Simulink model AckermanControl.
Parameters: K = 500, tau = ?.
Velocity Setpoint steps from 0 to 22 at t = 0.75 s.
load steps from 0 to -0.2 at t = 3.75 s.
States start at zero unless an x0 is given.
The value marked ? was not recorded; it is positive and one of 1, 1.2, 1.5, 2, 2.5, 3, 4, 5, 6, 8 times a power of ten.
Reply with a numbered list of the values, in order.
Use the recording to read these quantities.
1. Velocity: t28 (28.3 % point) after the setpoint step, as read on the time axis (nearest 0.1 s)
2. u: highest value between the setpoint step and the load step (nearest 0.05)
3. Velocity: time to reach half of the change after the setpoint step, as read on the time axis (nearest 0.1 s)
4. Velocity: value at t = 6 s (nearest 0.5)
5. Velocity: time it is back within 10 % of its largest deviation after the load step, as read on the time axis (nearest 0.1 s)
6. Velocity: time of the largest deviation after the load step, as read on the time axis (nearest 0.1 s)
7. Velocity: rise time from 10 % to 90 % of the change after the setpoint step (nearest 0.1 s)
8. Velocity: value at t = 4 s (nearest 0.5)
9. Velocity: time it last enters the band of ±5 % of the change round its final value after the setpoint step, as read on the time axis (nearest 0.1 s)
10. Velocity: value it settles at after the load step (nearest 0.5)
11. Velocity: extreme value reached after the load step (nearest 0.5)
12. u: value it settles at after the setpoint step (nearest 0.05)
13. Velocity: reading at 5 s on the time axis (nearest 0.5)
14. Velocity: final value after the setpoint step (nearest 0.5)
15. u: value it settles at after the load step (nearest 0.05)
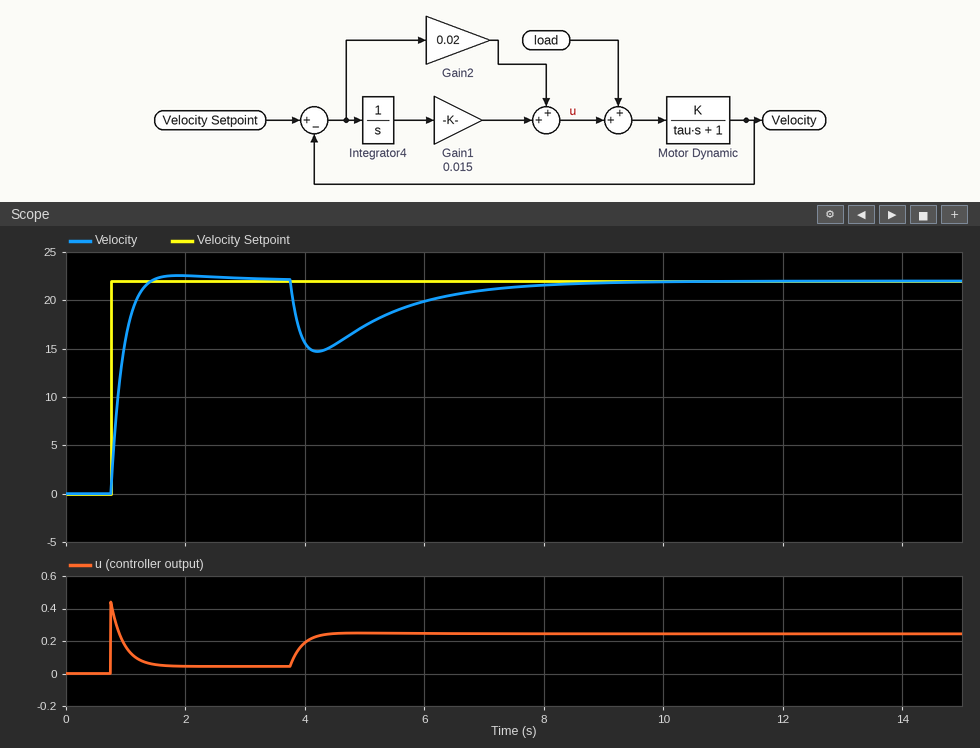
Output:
1. 0.8 s
2. 0.45
3. 0.9 s
4. 20.0
5. 7.3 s
6. 4.2 s
7. 0.4 s
8. 15.5
9. 1.3 s
10. 22.0
11. 14.5
12. 0.05
13. 17.5
14. 22.0
15. 0.25
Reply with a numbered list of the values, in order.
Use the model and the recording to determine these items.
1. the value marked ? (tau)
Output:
1. 2
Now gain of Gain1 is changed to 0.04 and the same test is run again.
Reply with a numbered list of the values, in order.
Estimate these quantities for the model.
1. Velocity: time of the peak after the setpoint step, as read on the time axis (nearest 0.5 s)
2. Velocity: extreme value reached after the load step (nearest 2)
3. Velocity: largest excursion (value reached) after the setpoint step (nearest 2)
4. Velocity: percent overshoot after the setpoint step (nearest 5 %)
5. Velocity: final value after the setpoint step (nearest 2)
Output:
1. 1.5 s
2. 16
3. 24
4. 10 %
5. 22
